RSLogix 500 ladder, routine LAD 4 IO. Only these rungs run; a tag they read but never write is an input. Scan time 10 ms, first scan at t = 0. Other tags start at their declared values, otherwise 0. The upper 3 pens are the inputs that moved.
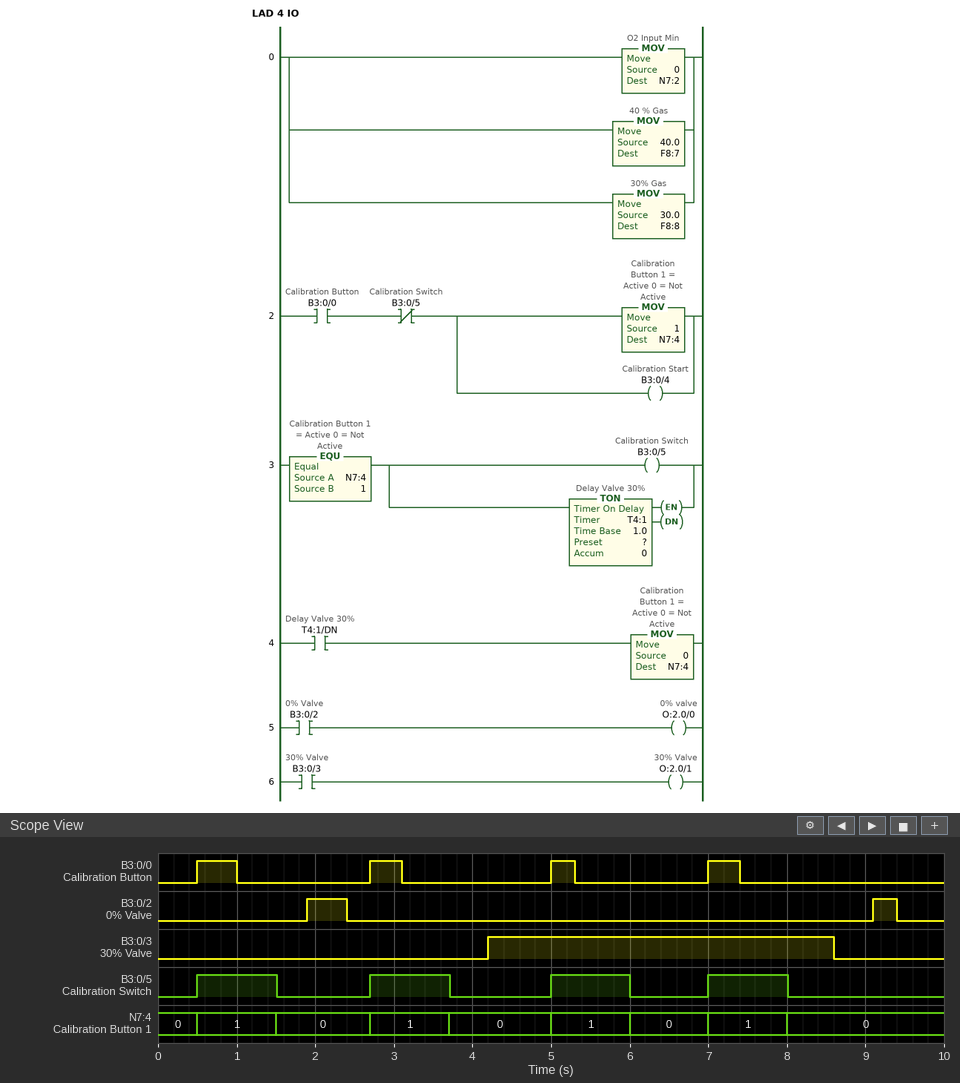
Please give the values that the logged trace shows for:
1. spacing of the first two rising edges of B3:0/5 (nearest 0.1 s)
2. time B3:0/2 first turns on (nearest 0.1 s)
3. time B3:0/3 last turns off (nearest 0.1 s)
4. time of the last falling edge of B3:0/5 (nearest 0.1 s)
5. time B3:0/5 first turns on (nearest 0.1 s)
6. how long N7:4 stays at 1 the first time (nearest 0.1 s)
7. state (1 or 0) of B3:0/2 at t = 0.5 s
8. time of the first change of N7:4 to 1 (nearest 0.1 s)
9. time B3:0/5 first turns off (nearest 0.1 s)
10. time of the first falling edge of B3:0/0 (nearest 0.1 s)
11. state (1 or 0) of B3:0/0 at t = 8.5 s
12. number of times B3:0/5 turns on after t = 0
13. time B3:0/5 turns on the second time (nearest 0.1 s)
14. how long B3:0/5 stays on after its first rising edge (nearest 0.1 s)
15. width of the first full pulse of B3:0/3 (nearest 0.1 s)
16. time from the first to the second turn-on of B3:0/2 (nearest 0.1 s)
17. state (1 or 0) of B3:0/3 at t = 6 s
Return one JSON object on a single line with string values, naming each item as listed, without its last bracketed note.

{"spacing of the first two rising edges of B3:0/5": "2.2 s", "time B3:0/2 first turns on": "1.9 s", "time B3:0/3 last turns off": "8.6 s", "time of the last falling edge of B3:0/5": "8.0 s", "time B3:0/5 first turns on": "0.5 s", "how long N7:4 stays at 1 the first time": "1.0 s", "state (1 or 0) of B3:0/2 at t = 0.5 s": "0", "time of the first change of N7:4 to 1": "0.5 s", "time B3:0/5 first turns off": "1.5 s", "time of the first falling edge of B3:0/0": "1.0 s", "state (1 or 0) of B3:0/0 at t = 8.5 s": "0", "number of times B3:0/5 turns on after t = 0": "4", "time B3:0/5 turns on the second time": "2.7 s", "how long B3:0/5 stays on after its first rising edge": "1.0 s", "width of the first full pulse of B3:0/3": "4.4 s", "time from the first to the second turn-on of B3:0/2": "7.2 s", "state (1 or 0) of B3:0/3 at t = 6 s": "1"}
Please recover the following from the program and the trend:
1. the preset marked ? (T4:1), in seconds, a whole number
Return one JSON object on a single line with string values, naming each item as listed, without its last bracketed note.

{"the preset marked ? (T4:1), in seconds, a whole number": "1 s"}
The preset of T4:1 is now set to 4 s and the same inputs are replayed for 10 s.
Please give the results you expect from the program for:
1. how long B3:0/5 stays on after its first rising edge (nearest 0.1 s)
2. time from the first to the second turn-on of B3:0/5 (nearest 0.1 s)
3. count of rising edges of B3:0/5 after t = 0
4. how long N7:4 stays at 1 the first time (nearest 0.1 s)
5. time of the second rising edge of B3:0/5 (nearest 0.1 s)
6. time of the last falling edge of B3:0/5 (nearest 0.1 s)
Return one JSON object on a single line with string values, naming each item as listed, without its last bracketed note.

{"how long B3:0/5 stays on after its first rising edge": "4.0 s", "time from the first to the second turn-on of B3:0/5": "4.5 s", "count of rising edges of B3:0/5 after t = 0": "2", "how long N7:4 stays at 1 the first time": "4.0 s", "time of the second rising edge of B3:0/5": "5.0 s", "time of the last falling edge of B3:0/5": "9.0 s"}
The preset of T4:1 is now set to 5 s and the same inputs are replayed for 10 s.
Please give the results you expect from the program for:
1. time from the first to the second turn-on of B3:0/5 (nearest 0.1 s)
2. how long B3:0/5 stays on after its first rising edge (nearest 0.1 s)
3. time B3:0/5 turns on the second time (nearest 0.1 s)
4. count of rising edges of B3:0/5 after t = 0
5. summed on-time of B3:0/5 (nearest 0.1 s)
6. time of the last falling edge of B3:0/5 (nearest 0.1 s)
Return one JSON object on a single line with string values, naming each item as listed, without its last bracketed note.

{"time from the first to the second turn-on of B3:0/5": "6.5 s", "how long B3:0/5 stays on after its first rising edge": "5.0 s", "time B3:0/5 turns on the second time": "7.0 s", "count of rising edges of B3:0/5 after t = 0": "2", "summed on-time of B3:0/5": "8.0 s", "time of the last falling edge of B3:0/5": "5.5 s"}
